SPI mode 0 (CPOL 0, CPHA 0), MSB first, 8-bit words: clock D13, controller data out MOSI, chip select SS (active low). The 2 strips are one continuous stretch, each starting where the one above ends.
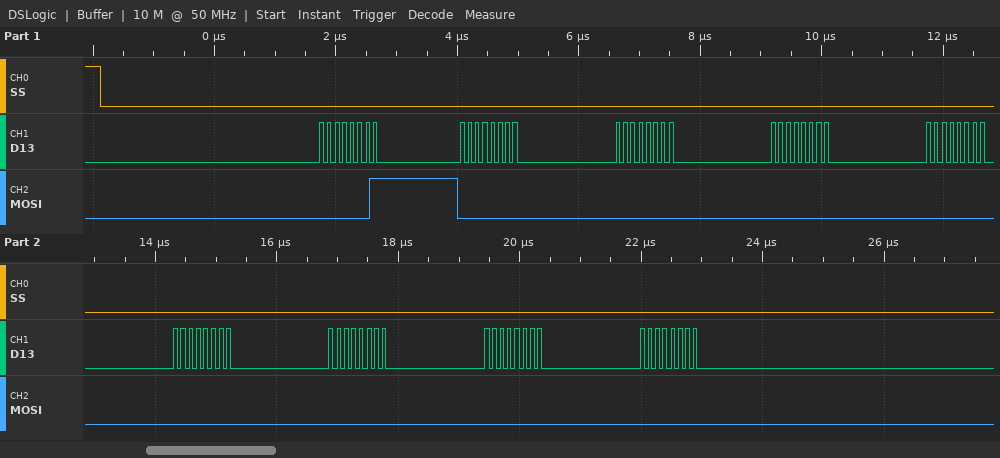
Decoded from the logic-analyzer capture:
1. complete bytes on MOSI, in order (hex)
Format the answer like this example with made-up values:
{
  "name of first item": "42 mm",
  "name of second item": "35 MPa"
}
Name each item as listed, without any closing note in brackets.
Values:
{
  "complete bytes on MOSI, in order": "01 00 00 00 00 00 00 00 00"
}
